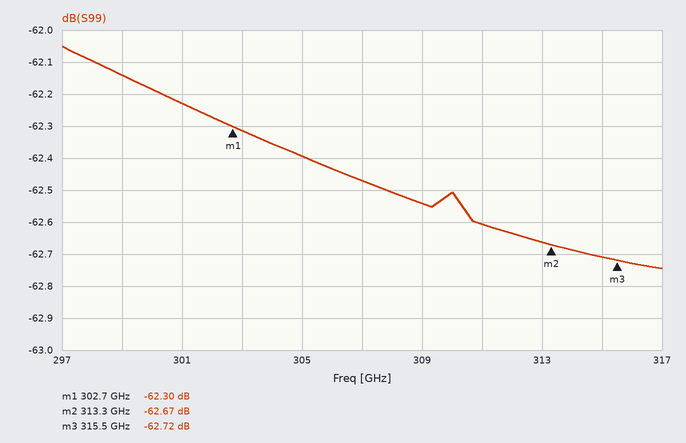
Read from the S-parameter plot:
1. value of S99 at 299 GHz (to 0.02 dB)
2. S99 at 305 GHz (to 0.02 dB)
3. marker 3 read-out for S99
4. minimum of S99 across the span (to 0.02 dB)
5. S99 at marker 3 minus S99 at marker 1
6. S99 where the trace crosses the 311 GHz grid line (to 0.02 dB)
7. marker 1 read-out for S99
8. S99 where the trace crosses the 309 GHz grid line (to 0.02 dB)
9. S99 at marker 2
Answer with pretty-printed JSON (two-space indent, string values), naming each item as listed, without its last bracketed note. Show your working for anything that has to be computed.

{
  "value of S99 at 299 GHz": "-62.14 dB",
  "S99 at 305 GHz": "-62.40 dB",
  "marker 3 read-out for S99": "-62.72 dB",
  "minimum of S99 across the span": "-62.74 dB",
  "S99 at marker 3 minus S99 at marker 1": "-62.72 − (-62.3) = -0.42 dB",
  "S99 where the trace crosses the 311 GHz grid line": "-62.60 dB",
  "marker 1 read-out for S99": "-62.30 dB",
  "S99 where the trace crosses the 309 GHz grid line": "-62.54 dB",
  "S99 at marker 2": "-62.67 dB"
}
